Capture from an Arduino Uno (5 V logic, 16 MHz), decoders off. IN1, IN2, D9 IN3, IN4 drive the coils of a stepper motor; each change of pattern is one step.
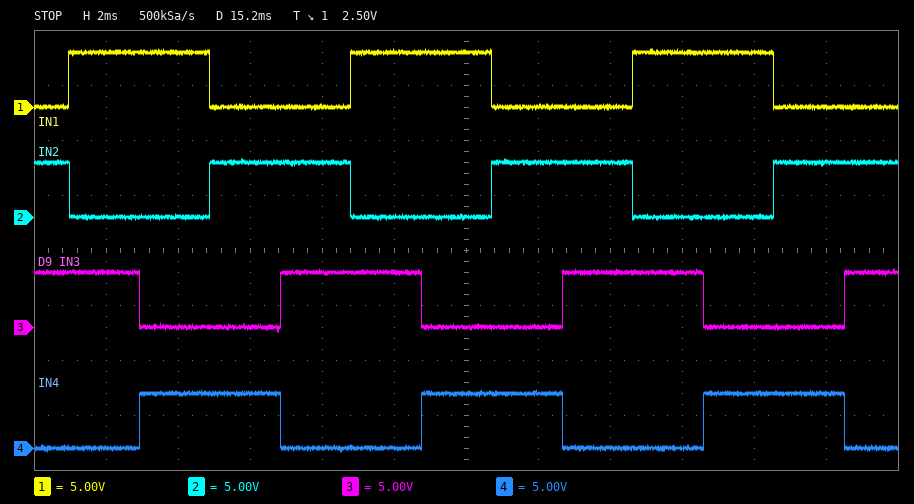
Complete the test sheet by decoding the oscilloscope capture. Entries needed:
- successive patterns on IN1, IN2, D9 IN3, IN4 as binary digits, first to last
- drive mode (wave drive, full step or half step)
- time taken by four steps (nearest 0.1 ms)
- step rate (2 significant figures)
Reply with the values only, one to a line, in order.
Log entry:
0110 1010 1001 0101 0110 1010 1001 0101 0110 1010 1001 0101 0110
full step
7.8 ms
510 steps/s
